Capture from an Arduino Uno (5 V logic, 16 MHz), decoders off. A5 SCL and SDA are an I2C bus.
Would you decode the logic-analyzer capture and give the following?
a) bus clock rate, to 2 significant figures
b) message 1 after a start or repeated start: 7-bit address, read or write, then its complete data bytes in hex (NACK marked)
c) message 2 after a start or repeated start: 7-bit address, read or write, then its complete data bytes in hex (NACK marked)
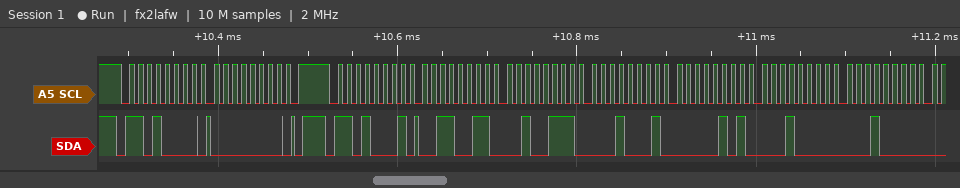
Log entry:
100 kHz
0x68 write: 00
0x68 read: 33 27 11 05 10 10
